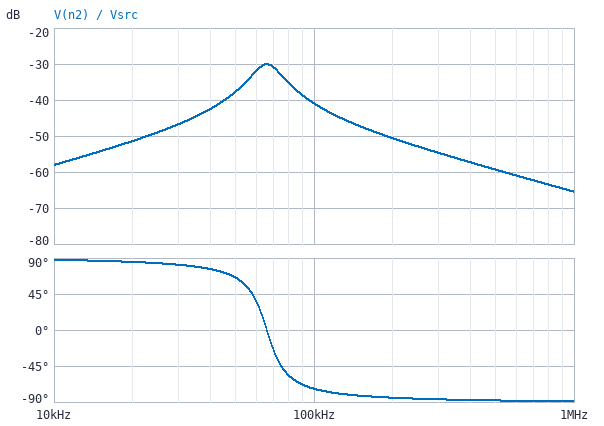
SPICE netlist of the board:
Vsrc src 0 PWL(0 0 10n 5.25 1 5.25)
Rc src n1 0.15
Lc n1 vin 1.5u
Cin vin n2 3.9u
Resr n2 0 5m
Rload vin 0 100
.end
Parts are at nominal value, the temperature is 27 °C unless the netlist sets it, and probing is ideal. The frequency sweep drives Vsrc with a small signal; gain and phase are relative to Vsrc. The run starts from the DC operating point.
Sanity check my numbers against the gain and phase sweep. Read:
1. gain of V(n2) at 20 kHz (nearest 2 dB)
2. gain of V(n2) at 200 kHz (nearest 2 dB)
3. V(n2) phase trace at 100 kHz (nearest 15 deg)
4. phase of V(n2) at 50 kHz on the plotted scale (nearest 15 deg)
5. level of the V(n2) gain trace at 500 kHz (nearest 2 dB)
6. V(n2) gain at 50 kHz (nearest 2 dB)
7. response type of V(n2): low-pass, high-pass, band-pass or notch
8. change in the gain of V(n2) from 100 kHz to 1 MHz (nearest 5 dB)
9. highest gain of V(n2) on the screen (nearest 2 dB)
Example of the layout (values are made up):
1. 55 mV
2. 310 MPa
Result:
1. -52 dB
2. -50 dB
3. -75 deg
4. 60 deg
5. -60 dB
6. -38 dB
7. band-pass
8. -25 dB
9. -30 dB
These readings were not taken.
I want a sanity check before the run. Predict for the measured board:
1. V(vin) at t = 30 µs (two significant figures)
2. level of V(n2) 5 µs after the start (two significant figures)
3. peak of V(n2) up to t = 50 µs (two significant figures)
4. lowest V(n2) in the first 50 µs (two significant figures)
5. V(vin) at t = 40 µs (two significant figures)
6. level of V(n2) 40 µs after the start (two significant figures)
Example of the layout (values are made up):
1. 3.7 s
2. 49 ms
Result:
1. 4.2 V
2. 29 mV
3. 35 mV
4. -23 mV
5. 5.8 V
6. -3.3 mV
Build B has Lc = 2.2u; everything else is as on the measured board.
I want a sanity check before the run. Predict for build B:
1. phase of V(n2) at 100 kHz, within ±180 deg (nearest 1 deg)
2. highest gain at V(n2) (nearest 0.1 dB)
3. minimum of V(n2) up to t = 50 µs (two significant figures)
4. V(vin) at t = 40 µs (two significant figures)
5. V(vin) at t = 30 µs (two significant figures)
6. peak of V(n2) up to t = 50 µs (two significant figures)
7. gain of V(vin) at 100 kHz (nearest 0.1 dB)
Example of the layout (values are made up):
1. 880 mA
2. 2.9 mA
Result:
1. -81 deg
2. -30.1 dB
3. -21 mV
4. 4.5 V
5. 6.6 V
6. 30 mV
7. -7.7 dB
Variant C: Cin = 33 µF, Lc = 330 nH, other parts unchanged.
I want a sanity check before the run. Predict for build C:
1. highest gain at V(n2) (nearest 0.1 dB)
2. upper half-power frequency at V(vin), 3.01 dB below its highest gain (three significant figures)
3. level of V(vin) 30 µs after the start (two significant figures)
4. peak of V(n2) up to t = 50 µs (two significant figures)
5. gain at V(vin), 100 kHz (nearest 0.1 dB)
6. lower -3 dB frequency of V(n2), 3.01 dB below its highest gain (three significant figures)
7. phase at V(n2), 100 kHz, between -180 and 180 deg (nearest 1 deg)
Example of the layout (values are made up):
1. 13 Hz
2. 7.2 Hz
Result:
1. -29.8 dB
2. 43.7 kHz
3. 5.2 V
4. 110 mV
5. -13.2 dB
6. 23.7 kHz
7. -46 deg
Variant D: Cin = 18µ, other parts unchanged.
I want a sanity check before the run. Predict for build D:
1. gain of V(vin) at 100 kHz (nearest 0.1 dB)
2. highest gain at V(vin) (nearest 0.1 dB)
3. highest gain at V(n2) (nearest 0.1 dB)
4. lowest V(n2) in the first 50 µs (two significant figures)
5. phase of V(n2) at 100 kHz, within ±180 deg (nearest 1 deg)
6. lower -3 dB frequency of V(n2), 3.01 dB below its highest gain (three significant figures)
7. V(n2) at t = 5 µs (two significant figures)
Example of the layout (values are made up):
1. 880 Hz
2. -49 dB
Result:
1. -19.8 dB
2. 5.7 dB
3. -29.9 dB
4. -26 mV
5. -80 deg
6. 23.5 kHz
7. 58 mV
